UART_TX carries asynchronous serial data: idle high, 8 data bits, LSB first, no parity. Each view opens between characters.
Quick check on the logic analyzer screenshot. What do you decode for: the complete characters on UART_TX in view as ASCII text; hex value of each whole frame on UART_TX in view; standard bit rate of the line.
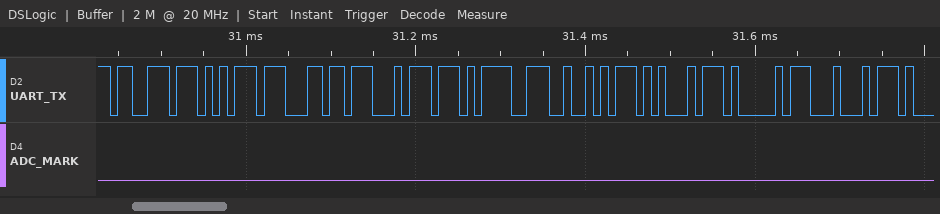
"sult=READ"
73, 75, 6C, 74, 3D, 52, 45, 41, 44
115200 baud
